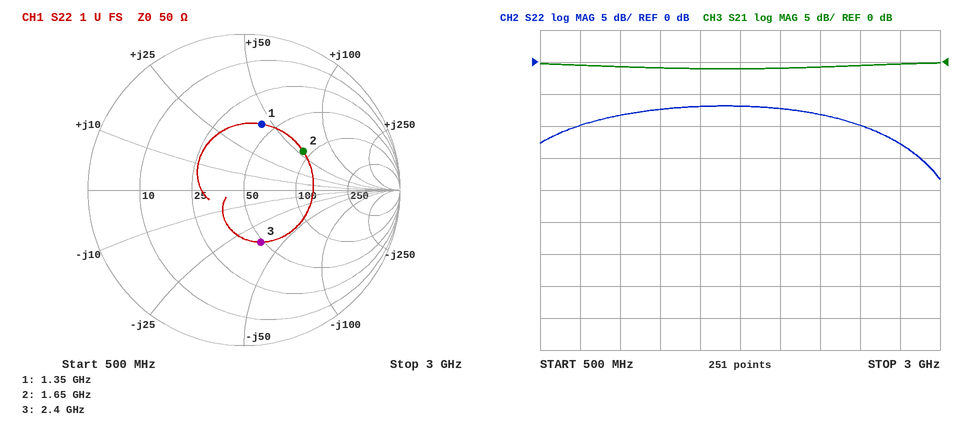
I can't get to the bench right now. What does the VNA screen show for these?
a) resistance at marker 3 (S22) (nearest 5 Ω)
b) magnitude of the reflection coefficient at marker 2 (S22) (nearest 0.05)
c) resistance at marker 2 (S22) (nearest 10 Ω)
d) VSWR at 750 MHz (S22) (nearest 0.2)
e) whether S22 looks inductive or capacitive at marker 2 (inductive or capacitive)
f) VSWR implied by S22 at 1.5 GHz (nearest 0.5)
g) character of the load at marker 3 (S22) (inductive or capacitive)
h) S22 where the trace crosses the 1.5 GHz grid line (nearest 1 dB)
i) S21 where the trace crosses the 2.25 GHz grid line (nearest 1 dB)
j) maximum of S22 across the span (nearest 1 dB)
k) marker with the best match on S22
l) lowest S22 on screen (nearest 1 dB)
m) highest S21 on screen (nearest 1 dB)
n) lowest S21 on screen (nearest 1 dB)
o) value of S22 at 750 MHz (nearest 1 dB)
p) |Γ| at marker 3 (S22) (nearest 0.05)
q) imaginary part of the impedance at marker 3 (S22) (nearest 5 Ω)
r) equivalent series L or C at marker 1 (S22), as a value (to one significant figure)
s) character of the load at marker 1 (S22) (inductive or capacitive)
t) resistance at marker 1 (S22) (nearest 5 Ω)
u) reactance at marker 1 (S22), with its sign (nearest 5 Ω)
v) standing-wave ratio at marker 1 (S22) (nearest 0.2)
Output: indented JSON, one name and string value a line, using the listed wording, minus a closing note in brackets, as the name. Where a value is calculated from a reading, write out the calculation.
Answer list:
{
  "resistance at marker 3 (S22)": "50 Ω",
  "magnitude of the reflection coefficient at marker 2 (S22)": "0.45",
  "resistance at marker 2 (S22)": "90 Ω",
  "VSWR at 750 MHz (S22)": "|Γ| = 10^(-10/20) = 0.3162; VSWR = (1 + 0.3162)/(1 − 0.3162) ≈ 1.92, so 2.0 to the nearest 0.2",
  "whether S22 looks inductive or capacitive at marker 2": "inductive",
  "VSWR implied by S22 at 1.5 GHz": "|Γ| = 10^(-7/20) = 0.4467; VSWR = (1 + 0.4467)/(1 − 0.4467) ≈ 2.61, so 2.5 to the nearest 0.5",
  "character of the load at marker 3 (S22)": "capacitive",
  "S22 where the trace crosses the 1.5 GHz grid line": "-7 dB",
  "S21 where the trace crosses the 2.25 GHz grid line": "-1 dB",
  "maximum of S22 across the span": "-7 dB",
  "marker with the best match on S22": "marker 3",
  "lowest S22 on screen": "-18 dB",
  "highest S21 on screen": "0 dB",
  "lowest S21 on screen": "-1 dB",
  "value of S22 at 750 MHz": "-10 dB",
  "|Γ| at marker 3 (S22)": "0.35",
  "imaginary part of the impedance at marker 3 (S22)": "-35 Ω",
  "equivalent series L or C at marker 1 (S22), as a value": "L = 45 Ω/(2π × 1.35 GHz) ≈ 5 nH",
  "character of the load at marker 1 (S22)": "inductive",
  "resistance at marker 1 (S22)": "40 Ω",
  "reactance at marker 1 (S22), with its sign": "+45 Ω",
  "standing-wave ratio at marker 1 (S22)": "2.6"
}
